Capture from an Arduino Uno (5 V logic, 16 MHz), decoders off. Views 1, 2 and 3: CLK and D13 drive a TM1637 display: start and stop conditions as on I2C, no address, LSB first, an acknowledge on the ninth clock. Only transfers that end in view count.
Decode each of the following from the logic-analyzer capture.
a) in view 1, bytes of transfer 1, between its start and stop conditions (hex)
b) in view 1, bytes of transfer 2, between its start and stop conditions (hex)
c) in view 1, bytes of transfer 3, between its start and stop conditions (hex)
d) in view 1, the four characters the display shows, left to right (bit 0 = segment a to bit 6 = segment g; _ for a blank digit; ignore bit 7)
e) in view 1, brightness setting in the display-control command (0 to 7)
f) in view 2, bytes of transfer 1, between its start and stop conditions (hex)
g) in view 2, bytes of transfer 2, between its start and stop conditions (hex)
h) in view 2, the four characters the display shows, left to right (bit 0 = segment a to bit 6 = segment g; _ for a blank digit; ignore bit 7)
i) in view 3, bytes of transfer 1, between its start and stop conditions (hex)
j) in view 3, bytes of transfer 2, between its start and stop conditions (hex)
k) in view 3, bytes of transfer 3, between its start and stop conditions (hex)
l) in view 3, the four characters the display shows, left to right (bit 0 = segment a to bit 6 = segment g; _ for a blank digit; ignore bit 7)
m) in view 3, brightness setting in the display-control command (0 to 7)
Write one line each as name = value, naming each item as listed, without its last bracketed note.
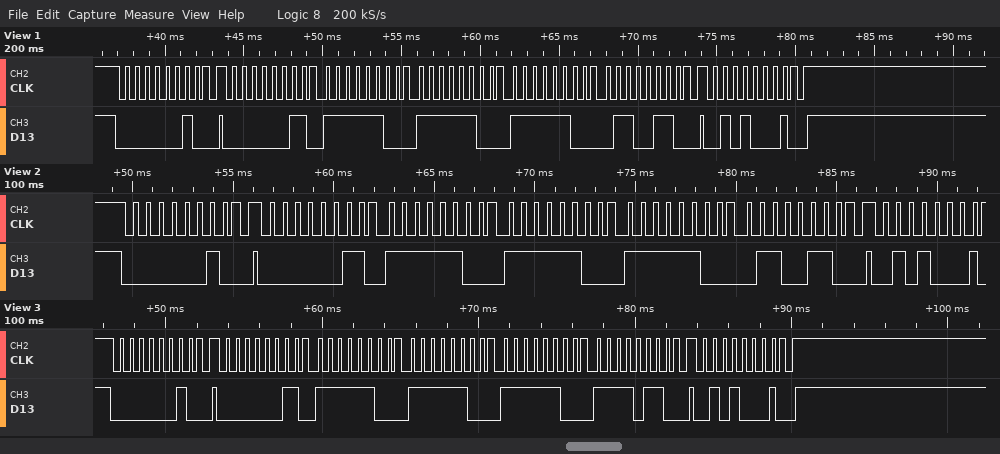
in view 1, bytes of transfer 1, between its start and stop conditions = 40
in view 1, bytes of transfer 2, between its start and stop conditions = C0 3F 3F 3F 66
in view 1, bytes of transfer 3, between its start and stop conditions = 8A
in view 1, the four characters the display shows, left to right = 0004
in view 1, brightness setting in the display-control command = 2
in view 2, bytes of transfer 1, between its start and stop conditions = 40
in view 2, bytes of transfer 2, between its start and stop conditions = C0 3F 3F 3F 66
in view 2, the four characters the display shows, left to right = 0004
in view 3, bytes of transfer 1, between its start and stop conditions = 40
in view 3, bytes of transfer 2, between its start and stop conditions = C0 3F 3F 3F 6F
in view 3, bytes of transfer 3, between its start and stop conditions = 8A
in view 3, the four characters the display shows, left to right = 0009
in view 3, brightness setting in the display-control command = 2
